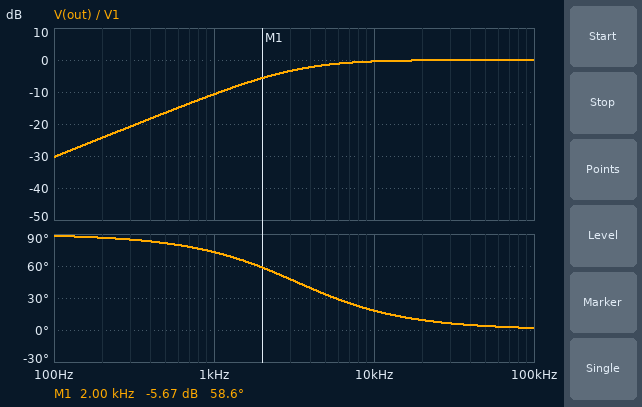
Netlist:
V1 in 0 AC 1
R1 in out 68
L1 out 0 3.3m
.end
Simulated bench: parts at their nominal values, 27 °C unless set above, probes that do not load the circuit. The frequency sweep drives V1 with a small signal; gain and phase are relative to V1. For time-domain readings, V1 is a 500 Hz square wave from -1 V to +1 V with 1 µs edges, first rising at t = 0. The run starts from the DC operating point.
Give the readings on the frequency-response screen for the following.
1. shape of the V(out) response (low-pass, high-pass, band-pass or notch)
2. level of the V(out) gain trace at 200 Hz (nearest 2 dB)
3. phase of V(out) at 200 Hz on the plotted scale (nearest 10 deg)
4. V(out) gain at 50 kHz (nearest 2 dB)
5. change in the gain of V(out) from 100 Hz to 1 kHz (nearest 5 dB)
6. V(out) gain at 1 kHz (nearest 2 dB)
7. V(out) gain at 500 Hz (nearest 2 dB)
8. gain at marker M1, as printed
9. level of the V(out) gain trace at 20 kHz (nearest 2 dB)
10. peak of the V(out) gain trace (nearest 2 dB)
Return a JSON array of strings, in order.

["high-pass", "-24 dB", "90 deg", "0 dB", "20 dB", "-10 dB", "-16 dB", "-5.67 dB", "0 dB", "0 dB"]
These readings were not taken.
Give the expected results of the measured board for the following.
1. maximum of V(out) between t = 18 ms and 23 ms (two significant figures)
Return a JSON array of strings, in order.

["2.0 V"]
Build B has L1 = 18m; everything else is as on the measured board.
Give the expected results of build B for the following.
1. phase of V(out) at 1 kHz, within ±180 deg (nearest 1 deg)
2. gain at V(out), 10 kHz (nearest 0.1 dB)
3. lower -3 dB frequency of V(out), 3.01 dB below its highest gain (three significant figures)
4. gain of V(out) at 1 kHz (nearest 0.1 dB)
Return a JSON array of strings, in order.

["31 deg", "0 dB", "601 Hz", "-1.3 dB"]
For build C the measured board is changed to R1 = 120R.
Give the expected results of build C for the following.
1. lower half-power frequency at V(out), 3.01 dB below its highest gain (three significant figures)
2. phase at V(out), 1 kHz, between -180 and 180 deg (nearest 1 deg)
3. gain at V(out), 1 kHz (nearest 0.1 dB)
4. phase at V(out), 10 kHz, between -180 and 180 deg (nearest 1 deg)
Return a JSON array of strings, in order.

["5.79 kHz", "80 deg", "-15.4 dB", "30 deg"]
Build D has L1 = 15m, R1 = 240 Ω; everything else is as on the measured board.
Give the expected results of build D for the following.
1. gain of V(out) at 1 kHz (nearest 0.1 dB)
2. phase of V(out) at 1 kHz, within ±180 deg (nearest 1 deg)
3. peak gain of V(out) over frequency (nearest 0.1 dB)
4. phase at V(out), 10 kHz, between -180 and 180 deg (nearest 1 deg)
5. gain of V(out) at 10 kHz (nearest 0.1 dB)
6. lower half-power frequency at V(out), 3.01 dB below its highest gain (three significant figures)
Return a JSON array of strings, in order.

["-8.7 dB", "69 deg", "0 dB", "14 deg", "-0.3 dB", "2.55 kHz"]
